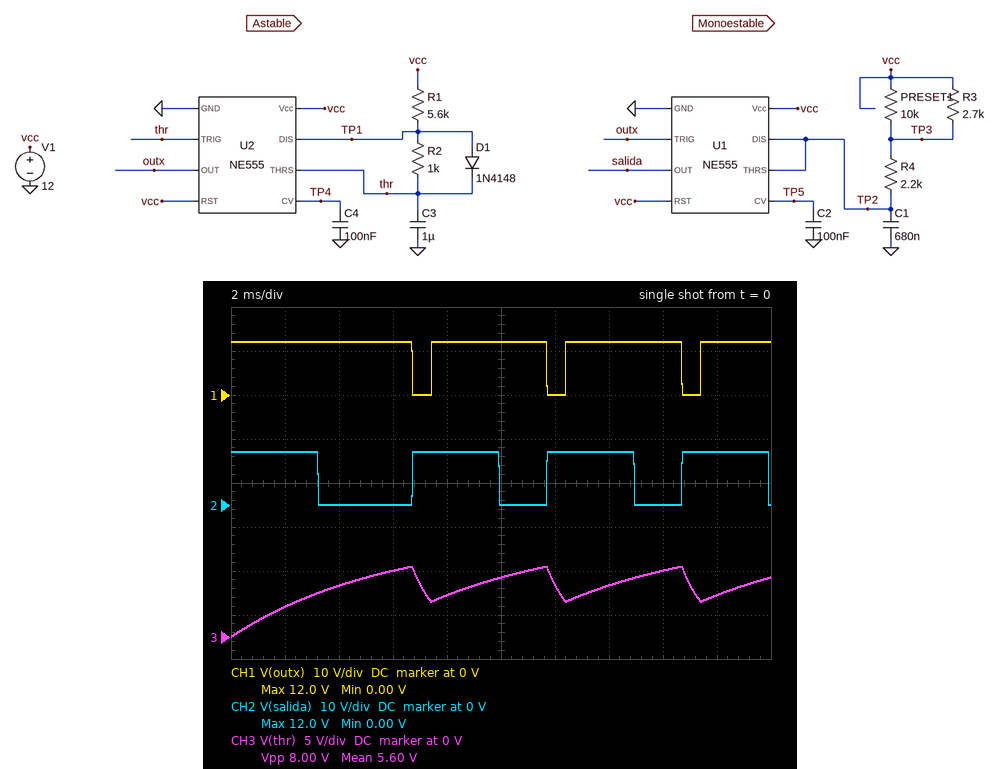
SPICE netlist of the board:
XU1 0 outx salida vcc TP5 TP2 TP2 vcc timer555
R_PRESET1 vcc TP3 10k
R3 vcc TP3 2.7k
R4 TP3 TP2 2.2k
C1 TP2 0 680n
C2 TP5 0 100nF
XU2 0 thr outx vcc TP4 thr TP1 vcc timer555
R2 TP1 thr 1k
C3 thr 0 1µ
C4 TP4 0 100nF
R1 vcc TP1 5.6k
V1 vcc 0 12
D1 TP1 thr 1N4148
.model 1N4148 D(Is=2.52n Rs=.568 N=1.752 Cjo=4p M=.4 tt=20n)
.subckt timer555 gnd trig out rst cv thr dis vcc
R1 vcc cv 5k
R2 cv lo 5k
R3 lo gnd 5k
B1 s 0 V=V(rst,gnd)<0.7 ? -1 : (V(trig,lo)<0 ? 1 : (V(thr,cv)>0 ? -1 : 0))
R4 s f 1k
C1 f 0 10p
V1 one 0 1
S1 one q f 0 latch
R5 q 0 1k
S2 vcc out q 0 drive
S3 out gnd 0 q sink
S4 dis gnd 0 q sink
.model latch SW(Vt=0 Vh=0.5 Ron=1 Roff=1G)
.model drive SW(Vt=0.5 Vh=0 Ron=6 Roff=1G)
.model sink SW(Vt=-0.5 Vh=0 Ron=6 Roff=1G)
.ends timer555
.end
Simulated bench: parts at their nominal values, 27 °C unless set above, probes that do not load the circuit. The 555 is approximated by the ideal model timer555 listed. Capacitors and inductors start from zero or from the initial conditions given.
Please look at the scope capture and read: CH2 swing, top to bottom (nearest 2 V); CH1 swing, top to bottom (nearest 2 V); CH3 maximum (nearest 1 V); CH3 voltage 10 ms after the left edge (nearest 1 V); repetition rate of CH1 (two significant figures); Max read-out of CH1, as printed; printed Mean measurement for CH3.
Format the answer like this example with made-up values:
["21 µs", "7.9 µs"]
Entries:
["12 V", "12 V", "8 V", "7 V", "200 Hz", "12.0 V", "5.60 V"]
